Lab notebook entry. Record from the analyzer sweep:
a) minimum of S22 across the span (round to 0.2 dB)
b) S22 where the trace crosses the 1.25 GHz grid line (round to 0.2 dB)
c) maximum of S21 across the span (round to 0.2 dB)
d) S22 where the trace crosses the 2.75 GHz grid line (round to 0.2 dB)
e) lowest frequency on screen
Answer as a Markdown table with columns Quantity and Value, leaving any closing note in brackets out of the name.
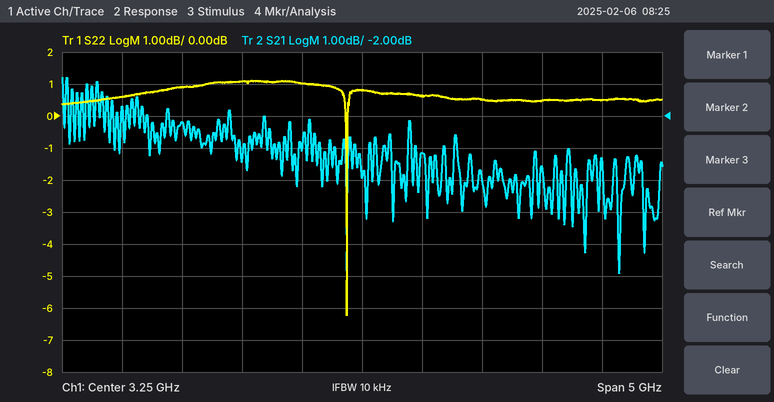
| Quantity | Value |
|---|---|
| minimum of S22 across the span | -6.2 dB |
| S22 where the trace crosses the 1.25 GHz grid line | 0.6 dB |
| maximum of S21 across the span | -0.8 dB |
| S22 where the trace crosses the 2.75 GHz grid line | 1.0 dB |
| lowest frequency on screen | 750 MHz |
